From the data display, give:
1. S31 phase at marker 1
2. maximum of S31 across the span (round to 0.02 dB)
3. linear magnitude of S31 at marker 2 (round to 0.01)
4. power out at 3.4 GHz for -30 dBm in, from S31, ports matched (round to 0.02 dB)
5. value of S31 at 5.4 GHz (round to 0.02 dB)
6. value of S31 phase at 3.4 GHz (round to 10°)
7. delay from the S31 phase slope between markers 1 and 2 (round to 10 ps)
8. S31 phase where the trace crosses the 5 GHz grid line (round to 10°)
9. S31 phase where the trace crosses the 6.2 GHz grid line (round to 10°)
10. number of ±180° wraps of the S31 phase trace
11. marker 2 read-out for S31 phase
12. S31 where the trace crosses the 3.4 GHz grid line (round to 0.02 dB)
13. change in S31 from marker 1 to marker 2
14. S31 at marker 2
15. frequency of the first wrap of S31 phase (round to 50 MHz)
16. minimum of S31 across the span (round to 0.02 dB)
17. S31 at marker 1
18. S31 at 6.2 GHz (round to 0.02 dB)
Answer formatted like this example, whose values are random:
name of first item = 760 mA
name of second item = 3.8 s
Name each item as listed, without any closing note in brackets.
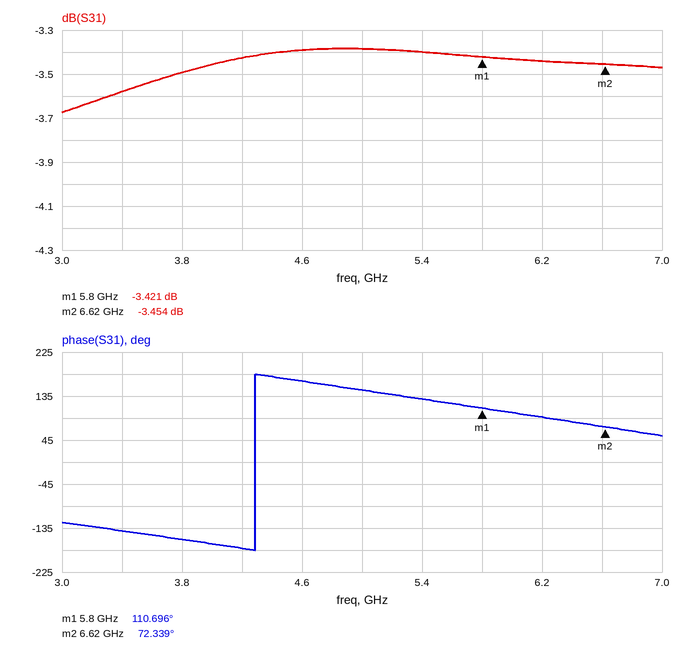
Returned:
S31 phase at marker 1 = 110.696°
maximum of S31 across the span = -3.38 dB
linear magnitude of S31 at marker 2 = 0.67
power out at 3.4 GHz for -30 dBm in, from S31, ports matched = -33.58 dBm
value of S31 at 5.4 GHz = -3.40 dB
value of S31 phase at 3.4 GHz = -140°
delay from the S31 phase slope between markers 1 and 2 = 130 ps
S31 phase where the trace crosses the 5 GHz grid line = 150°
S31 phase where the trace crosses the 6.2 GHz grid line = 90°
number of ±180° wraps of the S31 phase trace = 1
marker 2 read-out for S31 phase = 72.339°
S31 where the trace crosses the 3.4 GHz grid line = -3.58 dB
change in S31 from marker 1 to marker 2 = -0.033 dB
S31 at marker 2 = -3.454 dB
frequency of the first wrap of S31 phase = 4.30 GHz
minimum of S31 across the span = -3.68 dB
S31 at marker 1 = -3.421 dB
S31 at 6.2 GHz = -3.44 dB
